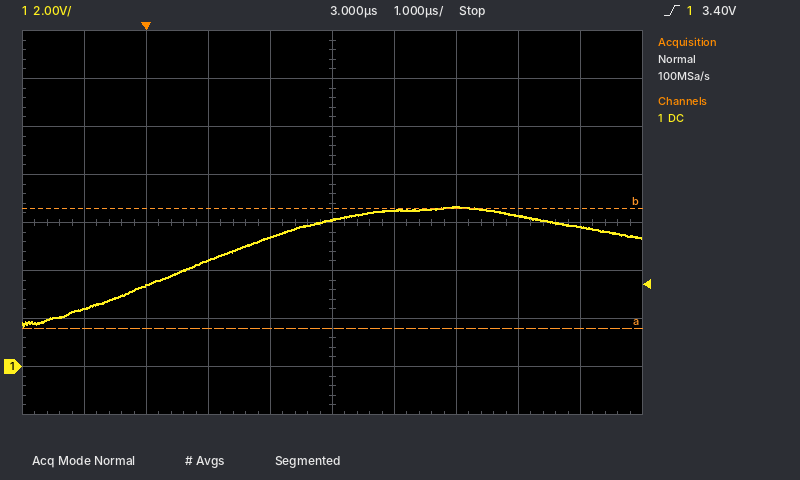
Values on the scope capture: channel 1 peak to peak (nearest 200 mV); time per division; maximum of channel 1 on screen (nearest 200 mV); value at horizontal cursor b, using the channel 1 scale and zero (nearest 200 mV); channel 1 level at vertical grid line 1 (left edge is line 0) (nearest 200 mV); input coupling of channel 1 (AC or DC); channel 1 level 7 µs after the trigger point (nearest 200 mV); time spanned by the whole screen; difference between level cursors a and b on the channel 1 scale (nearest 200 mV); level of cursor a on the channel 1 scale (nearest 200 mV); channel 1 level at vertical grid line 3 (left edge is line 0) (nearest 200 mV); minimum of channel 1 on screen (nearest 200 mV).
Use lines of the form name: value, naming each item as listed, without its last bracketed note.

channel 1 peak to peak: 5.0 V
time per division: 1 µs
maximum of channel 1 on screen: 6.6 V
value at horizontal cursor b, using the channel 1 scale and zero: 6.6 V
channel 1 level at vertical grid line 1 (left edge is line 0): 2.4 V
input coupling of channel 1: DC
channel 1 level 7 µs after the trigger point: 5.8 V
time spanned by the whole screen: 10 µs
difference between level cursors a and b on the channel 1 scale: 5.0 V
level of cursor a on the channel 1 scale: 1.6 V
channel 1 level at vertical grid line 3 (left edge is line 0): 4.4 V
minimum of channel 1 on screen: 1.6 V
